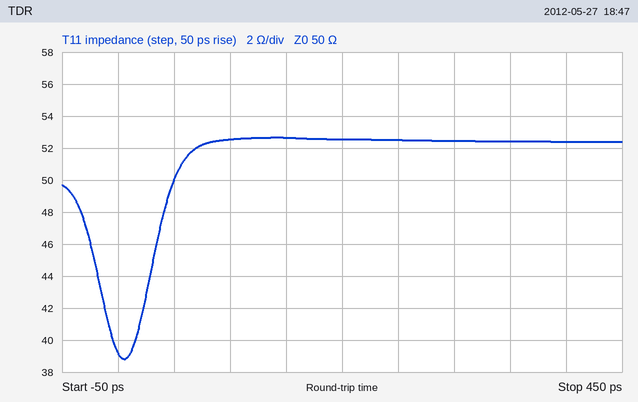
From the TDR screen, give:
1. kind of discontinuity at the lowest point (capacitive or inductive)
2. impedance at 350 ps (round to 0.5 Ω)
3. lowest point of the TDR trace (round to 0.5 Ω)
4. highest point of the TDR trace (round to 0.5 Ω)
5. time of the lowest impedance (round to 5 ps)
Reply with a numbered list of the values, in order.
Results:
1. capacitive
2. 52.5 Ω
3. 39.0 Ω
4. 52.5 Ω
5. 5 ps
